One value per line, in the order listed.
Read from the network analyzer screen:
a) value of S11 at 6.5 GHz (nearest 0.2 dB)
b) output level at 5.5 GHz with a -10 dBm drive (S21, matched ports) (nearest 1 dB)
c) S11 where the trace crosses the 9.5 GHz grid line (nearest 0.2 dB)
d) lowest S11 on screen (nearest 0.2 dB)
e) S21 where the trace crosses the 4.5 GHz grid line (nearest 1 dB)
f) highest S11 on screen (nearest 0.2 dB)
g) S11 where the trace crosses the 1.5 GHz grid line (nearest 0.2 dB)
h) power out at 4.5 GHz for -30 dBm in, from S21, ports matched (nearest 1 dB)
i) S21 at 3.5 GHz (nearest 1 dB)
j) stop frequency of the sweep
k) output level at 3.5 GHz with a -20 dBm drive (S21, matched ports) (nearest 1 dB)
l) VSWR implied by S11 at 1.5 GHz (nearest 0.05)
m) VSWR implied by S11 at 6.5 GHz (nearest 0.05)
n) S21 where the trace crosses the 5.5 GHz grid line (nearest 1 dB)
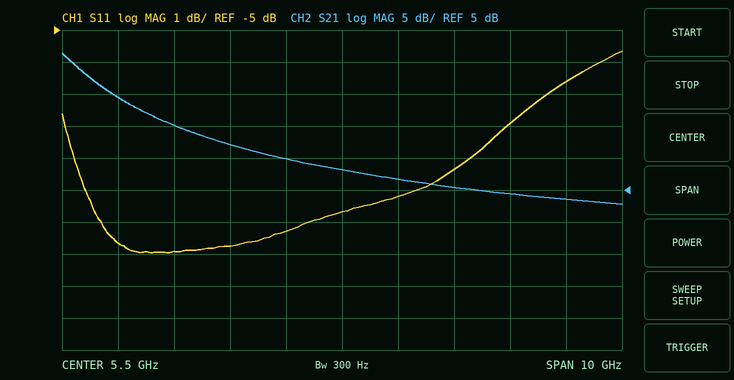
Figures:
-10.2 dB
-2 dBm
-6.6 dB
-12.0 dB
10 dB
-5.6 dB
-11.6 dB
-20 dBm
12 dB
10.5 GHz
-8 dBm
1.70
1.90
8 dB
